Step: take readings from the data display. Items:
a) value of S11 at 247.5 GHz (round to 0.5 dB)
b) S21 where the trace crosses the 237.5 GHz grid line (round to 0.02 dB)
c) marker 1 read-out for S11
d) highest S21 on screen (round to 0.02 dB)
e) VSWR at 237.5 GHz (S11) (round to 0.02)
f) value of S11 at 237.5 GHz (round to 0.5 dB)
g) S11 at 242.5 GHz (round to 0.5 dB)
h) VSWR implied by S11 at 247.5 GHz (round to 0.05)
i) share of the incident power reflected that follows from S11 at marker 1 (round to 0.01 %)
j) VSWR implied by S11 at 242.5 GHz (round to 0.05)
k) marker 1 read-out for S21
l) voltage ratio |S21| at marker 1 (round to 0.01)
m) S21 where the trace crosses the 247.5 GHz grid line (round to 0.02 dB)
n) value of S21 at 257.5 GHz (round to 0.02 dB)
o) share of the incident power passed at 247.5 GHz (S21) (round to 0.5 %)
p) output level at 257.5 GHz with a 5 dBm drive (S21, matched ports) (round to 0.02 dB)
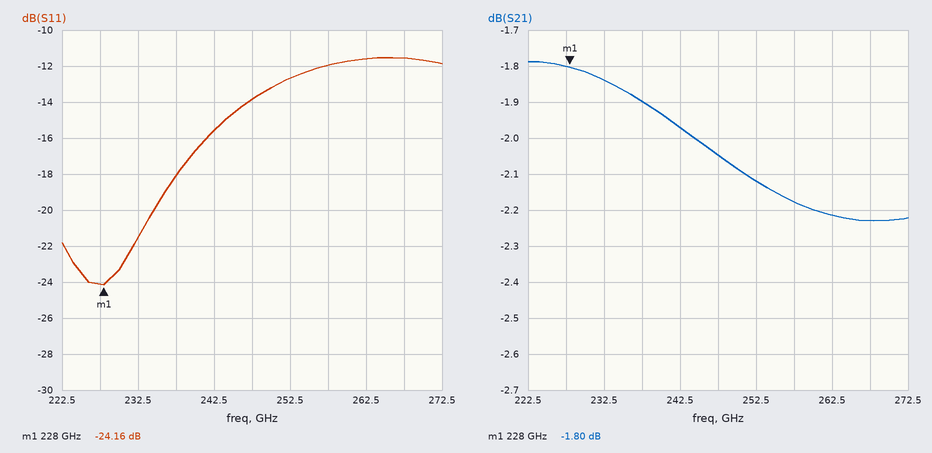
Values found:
-14.0 dB
-1.90 dB
-24.16 dB
-1.78 dB
1.28
-18.0 dB
-15.5 dB
1.50
0.38 %
1.40
-1.80 dB
0.81
-2.04 dB
-2.18 dB
62.5 %
2.82 dBm
